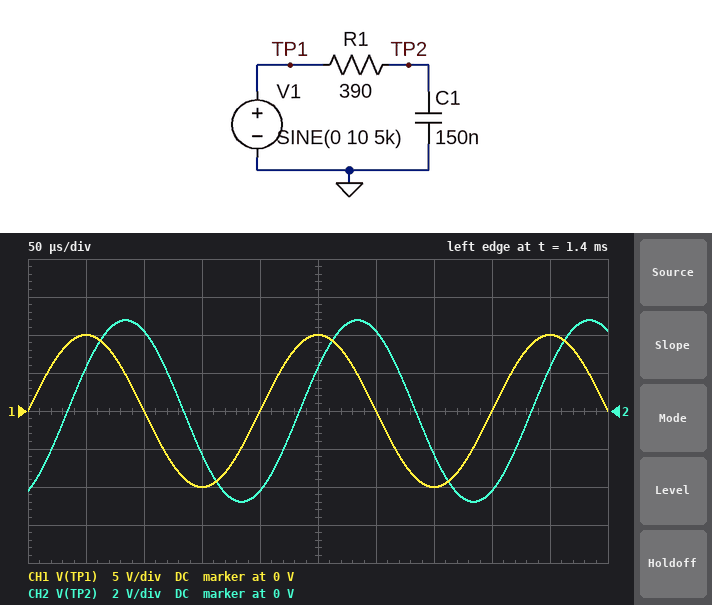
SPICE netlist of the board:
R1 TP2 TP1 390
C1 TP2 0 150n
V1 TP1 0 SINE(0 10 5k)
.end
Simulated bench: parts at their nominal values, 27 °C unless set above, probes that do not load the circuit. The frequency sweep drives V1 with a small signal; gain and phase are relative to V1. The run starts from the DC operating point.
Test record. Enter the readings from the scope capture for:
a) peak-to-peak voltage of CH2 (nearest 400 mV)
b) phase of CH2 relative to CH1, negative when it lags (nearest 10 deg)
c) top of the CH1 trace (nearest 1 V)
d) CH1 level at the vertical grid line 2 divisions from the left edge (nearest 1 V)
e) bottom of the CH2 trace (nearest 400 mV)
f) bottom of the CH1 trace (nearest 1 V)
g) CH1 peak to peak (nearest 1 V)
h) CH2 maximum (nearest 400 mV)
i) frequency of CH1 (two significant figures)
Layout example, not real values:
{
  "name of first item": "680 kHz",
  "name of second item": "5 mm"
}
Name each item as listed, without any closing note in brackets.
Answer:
{
  "peak-to-peak voltage of CH2": "9.6 V",
  "phase of CH2 relative to CH1, negative when it lags": "-60 deg",
  "top of the CH1 trace": "10 V",
  "CH1 level at the vertical grid line 2 divisions from the left edge": "0 V",
  "bottom of the CH2 trace": "-4.8 V",
  "bottom of the CH1 trace": "-10 V",
  "CH1 peak to peak": "20 V",
  "CH2 maximum": "4.8 V",
  "frequency of CH1": "5.0 kHz"
}
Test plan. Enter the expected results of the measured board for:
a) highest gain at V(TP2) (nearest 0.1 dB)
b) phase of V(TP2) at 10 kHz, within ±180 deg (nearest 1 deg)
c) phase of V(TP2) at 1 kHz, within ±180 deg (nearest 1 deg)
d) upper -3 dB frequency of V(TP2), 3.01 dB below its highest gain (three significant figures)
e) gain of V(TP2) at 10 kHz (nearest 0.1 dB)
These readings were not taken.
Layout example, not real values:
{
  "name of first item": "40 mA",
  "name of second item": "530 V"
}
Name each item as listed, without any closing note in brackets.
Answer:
{
  "highest gain at V(TP2)": "0 dB",
  "phase of V(TP2) at 10 kHz, within ±180 deg": "-75 deg",
  "phase of V(TP2) at 1 kHz, within ±180 deg": "-20 deg",
  "upper -3 dB frequency of V(TP2), 3.01 dB below its highest gain": "2.72 kHz",
  "gain of V(TP2) at 10 kHz": "-11.6 dB"
}
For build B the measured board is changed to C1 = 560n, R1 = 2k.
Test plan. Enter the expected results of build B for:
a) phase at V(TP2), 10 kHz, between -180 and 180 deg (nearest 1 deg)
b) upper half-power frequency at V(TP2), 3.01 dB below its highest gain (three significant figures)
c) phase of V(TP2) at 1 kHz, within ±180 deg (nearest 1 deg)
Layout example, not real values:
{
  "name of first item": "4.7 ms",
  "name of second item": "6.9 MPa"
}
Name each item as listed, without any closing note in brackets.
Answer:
{
  "phase at V(TP2), 10 kHz, between -180 and 180 deg": "-89 deg",
  "upper half-power frequency at V(TP2), 3.01 dB below its highest gain": "142 Hz",
  "phase of V(TP2) at 1 kHz, within ±180 deg": "-82 deg"
}
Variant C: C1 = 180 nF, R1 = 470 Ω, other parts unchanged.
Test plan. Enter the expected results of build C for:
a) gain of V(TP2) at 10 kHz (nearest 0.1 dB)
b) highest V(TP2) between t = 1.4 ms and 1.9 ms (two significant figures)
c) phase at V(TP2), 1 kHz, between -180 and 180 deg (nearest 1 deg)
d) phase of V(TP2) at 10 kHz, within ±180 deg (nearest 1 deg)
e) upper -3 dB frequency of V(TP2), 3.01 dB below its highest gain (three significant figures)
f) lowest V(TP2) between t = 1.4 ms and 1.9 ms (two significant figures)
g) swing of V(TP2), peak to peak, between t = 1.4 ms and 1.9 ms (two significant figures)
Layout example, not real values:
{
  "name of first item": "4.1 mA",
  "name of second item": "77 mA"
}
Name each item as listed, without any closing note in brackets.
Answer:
{
  "gain of V(TP2) at 10 kHz": "-14.7 dB",
  "highest V(TP2) between t = 1.4 ms and 1.9 ms": "3.5 V",
  "phase at V(TP2), 1 kHz, between -180 and 180 deg": "-28 deg",
  "phase of V(TP2) at 10 kHz, within ±180 deg": "-79 deg",
  "upper -3 dB frequency of V(TP2), 3.01 dB below its highest gain": "1.88 kHz",
  "lowest V(TP2) between t = 1.4 ms and 1.9 ms": "-3.5 V",
  "swing of V(TP2), peak to peak, between t = 1.4 ms and 1.9 ms": "7.0 V"
}
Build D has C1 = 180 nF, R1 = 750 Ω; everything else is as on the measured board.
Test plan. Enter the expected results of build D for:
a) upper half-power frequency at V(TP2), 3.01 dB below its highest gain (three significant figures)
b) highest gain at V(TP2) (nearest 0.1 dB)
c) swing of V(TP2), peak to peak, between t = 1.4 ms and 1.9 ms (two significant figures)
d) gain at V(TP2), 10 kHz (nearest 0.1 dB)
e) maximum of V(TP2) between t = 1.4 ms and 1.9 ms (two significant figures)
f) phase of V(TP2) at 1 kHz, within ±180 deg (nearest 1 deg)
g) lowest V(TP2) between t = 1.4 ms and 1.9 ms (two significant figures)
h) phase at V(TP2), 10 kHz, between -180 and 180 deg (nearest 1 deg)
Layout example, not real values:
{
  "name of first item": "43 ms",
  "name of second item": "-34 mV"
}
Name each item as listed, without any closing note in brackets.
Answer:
{
  "upper half-power frequency at V(TP2), 3.01 dB below its highest gain": "1.18 kHz",
  "highest gain at V(TP2)": "0 dB",
  "swing of V(TP2), peak to peak, between t = 1.4 ms and 1.9 ms": "4.6 V",
  "gain at V(TP2), 10 kHz": "-18.6 dB",
  "maximum of V(TP2) between t = 1.4 ms and 1.9 ms": "2.3 V",
  "phase of V(TP2) at 1 kHz, within ±180 deg": "-40 deg",
  "lowest V(TP2) between t = 1.4 ms and 1.9 ms": "-2.3 V",
  "phase at V(TP2), 10 kHz, between -180 and 180 deg": "-83 deg"
}
